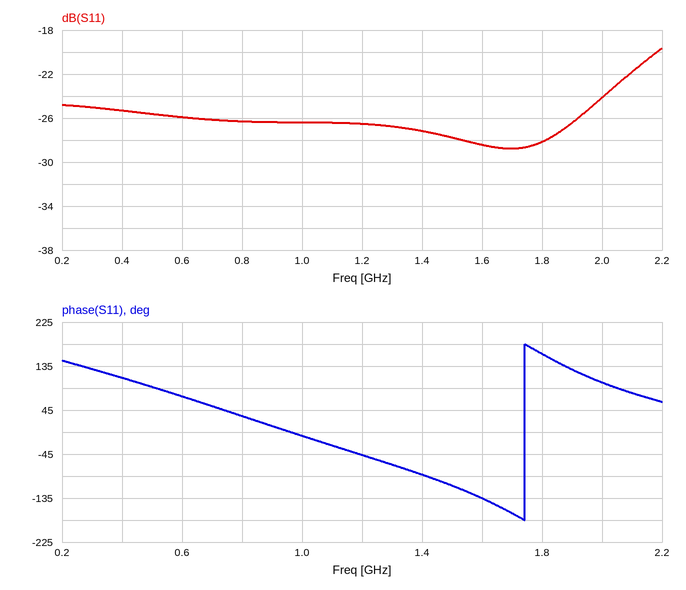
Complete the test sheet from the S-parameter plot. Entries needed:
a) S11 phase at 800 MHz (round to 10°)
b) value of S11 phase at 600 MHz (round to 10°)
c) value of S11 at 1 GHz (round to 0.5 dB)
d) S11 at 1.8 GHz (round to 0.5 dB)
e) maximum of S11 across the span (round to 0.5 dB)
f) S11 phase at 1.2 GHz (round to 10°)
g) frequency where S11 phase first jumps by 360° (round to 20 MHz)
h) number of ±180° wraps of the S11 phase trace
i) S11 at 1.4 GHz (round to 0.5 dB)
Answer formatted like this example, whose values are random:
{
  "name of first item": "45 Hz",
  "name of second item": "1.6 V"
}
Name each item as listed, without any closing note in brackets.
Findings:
{
  "S11 phase at 800 MHz": "30°",
  "value of S11 phase at 600 MHz": "70°",
  "value of S11 at 1 GHz": "-26.5 dB",
  "S11 at 1.8 GHz": "-28.0 dB",
  "maximum of S11 across the span": "-19.5 dB",
  "S11 phase at 1.2 GHz": "-50°",
  "frequency where S11 phase first jumps by 360°": "1.74 GHz",
  "number of ±180° wraps of the S11 phase trace": "1",
  "S11 at 1.4 GHz": "-27.0 dB"
}
